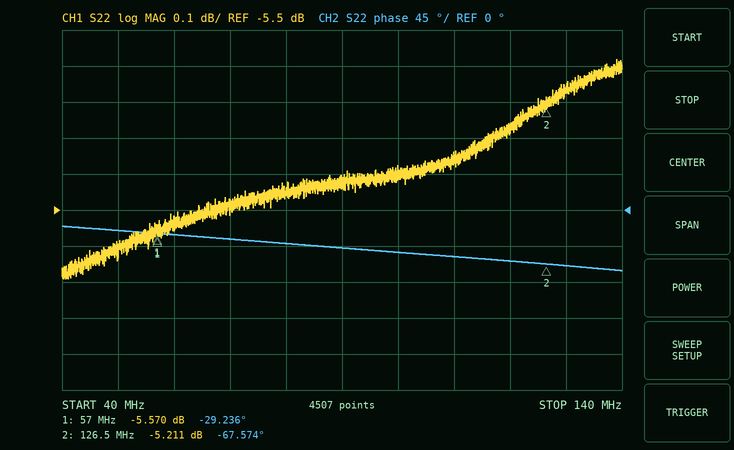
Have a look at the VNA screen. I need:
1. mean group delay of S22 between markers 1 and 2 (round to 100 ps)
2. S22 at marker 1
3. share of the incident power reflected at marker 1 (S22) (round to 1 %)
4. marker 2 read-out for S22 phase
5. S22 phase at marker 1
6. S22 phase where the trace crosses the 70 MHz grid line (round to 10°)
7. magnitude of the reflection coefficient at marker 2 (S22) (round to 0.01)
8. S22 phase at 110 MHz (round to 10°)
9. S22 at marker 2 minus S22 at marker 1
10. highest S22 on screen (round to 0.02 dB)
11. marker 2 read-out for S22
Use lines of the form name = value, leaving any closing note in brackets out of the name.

mean group delay of S22 between markers 1 and 2 = 1.5 ns
S22 at marker 1 = -5.570 dB
share of the incident power reflected at marker 1 (S22) = 28 %
marker 2 read-out for S22 phase = -67.574°
S22 phase at marker 1 = -29.236°
S22 phase where the trace crosses the 70 MHz grid line = -40°
magnitude of the reflection coefficient at marker 2 (S22) = 0.55
S22 phase at 110 MHz = -60°
S22 at marker 2 minus S22 at marker 1 = 0.359 dB
highest S22 on screen = -5.08 dB
marker 2 read-out for S22 = -5.211 dB
